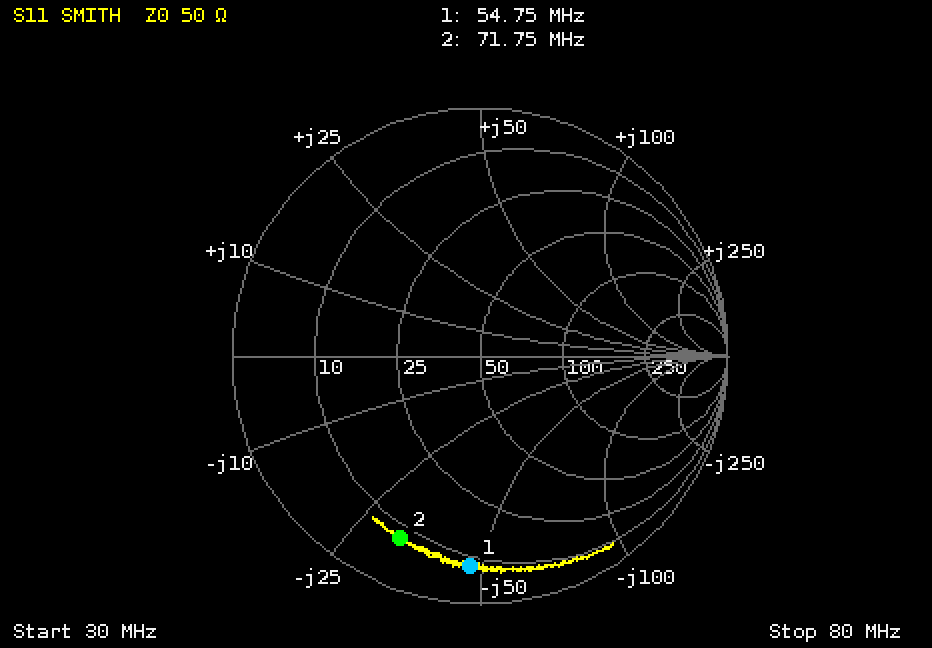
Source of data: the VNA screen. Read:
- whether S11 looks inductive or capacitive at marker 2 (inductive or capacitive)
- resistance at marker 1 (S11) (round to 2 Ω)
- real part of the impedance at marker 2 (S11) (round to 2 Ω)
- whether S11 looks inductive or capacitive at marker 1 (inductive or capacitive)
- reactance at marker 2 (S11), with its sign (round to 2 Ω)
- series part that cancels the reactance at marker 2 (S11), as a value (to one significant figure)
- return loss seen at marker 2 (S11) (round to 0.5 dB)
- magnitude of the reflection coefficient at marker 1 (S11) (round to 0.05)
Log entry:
capacitive
8 Ω
8 Ω
capacitive
-32 Ω
70 nH
2.0 dB
0.85
